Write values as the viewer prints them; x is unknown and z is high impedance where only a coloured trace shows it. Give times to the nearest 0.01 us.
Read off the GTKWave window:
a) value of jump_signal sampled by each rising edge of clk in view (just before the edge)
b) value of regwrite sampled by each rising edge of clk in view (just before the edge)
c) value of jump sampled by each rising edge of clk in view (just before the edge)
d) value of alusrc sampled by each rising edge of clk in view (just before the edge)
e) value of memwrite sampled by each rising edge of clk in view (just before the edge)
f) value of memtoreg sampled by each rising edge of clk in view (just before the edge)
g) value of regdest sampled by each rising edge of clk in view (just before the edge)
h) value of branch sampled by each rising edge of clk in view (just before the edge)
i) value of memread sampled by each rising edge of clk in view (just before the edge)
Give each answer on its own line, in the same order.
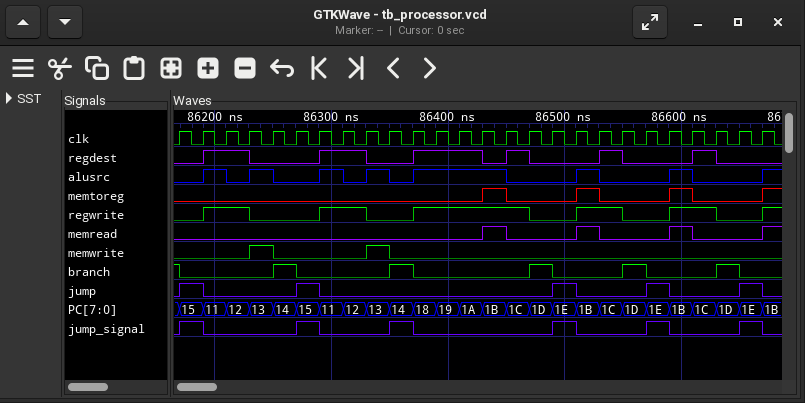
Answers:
0 1 0 0 0 0 1 0 0 0 1 0 0 0 0 0 0 1 0 0 0 1 0 0 0 1
0 0 1 1 0 0 0 1 1 0 0 1 1 1 1 1 0 0 1 1 0 0 1 1 0 0
0 1 0 0 0 0 1 0 0 0 0 0 0 0 0 0 0 1 0 0 0 1 0 0 0 1
0 0 1 0 1 0 0 1 0 1 0 1 1 1 1 0 0 0 1 0 0 0 1 0 0 0
0 0 0 0 1 0 0 0 0 1 0 0 0 0 0 0 0 0 0 0 0 0 0 0 0 0
0 0 0 0 0 0 0 0 0 0 0 0 0 0 1 0 0 0 1 0 0 0 1 0 0 0
0 0 1 1 0 0 0 1 1 0 0 1 1 1 0 1 0 0 0 1 0 0 0 1 0 0
1 0 0 0 0 1 0 0 0 0 1 0 0 0 0 0 1 0 0 0 1 0 0 0 1 0
0 0 0 0 0 0 0 0 0 0 0 0 0 0 1 0 0 0 1 0 0 0 1 0 0 0
